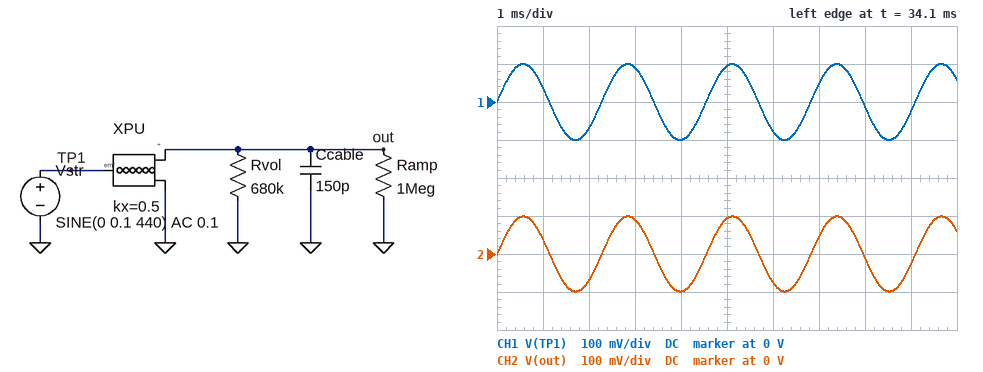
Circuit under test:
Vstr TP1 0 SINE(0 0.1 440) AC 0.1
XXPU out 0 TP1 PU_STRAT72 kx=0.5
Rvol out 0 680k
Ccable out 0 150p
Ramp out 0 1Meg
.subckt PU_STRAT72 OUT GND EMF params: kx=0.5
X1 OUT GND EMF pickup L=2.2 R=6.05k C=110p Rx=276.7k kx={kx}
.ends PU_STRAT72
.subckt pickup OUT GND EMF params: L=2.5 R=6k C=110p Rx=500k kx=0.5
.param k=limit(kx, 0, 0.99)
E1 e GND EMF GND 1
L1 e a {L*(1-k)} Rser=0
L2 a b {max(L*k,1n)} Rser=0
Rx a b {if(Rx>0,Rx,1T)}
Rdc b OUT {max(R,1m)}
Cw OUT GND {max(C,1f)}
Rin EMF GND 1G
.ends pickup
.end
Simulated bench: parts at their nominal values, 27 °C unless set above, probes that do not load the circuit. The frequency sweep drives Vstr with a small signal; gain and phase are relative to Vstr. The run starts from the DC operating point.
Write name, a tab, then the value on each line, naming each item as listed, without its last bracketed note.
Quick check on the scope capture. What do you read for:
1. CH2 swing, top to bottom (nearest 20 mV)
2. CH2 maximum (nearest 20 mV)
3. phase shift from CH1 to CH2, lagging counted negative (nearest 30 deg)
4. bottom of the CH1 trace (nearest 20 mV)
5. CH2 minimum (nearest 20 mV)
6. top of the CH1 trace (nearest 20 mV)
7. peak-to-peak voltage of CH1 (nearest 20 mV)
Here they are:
CH2 swing, top to bottom	200 mV
CH2 maximum	100 mV
phase shift from CH1 to CH2, lagging counted negative	0 deg
bottom of the CH1 trace	-100 mV
CH2 minimum	-100 mV
top of the CH1 trace	100 mV
peak-to-peak voltage of CH1	200 mV
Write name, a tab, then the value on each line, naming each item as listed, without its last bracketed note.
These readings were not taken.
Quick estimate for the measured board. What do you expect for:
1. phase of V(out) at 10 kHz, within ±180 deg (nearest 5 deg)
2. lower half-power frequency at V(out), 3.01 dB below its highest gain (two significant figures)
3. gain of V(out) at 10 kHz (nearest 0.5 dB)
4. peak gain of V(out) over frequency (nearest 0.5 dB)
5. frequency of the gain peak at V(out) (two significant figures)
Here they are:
phase of V(out) at 10 kHz, within ±180 deg	-150 deg
lower half-power frequency at V(out), 3.01 dB below its highest gain	5.0 kHz
gain of V(out) at 10 kHz	-2.5 dB
peak gain of V(out) over frequency	8.5 dB
frequency of the gain peak at V(out)	6.5 kHz
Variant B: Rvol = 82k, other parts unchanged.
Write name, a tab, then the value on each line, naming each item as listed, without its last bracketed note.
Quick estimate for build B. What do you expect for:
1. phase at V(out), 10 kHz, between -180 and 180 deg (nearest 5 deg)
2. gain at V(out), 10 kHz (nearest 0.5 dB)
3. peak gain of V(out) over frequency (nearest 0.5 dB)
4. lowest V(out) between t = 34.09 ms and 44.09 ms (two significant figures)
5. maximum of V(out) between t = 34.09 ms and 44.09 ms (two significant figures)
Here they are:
phase at V(out), 10 kHz, between -180 and 180 deg	-115 deg
gain at V(out), 10 kHz	-7.5 dB
peak gain of V(out) over frequency	-0.5 dB
lowest V(out) between t = 34.09 ms and 44.09 ms	-93 mV
maximum of V(out) between t = 34.09 ms and 44.09 ms	93 mV
